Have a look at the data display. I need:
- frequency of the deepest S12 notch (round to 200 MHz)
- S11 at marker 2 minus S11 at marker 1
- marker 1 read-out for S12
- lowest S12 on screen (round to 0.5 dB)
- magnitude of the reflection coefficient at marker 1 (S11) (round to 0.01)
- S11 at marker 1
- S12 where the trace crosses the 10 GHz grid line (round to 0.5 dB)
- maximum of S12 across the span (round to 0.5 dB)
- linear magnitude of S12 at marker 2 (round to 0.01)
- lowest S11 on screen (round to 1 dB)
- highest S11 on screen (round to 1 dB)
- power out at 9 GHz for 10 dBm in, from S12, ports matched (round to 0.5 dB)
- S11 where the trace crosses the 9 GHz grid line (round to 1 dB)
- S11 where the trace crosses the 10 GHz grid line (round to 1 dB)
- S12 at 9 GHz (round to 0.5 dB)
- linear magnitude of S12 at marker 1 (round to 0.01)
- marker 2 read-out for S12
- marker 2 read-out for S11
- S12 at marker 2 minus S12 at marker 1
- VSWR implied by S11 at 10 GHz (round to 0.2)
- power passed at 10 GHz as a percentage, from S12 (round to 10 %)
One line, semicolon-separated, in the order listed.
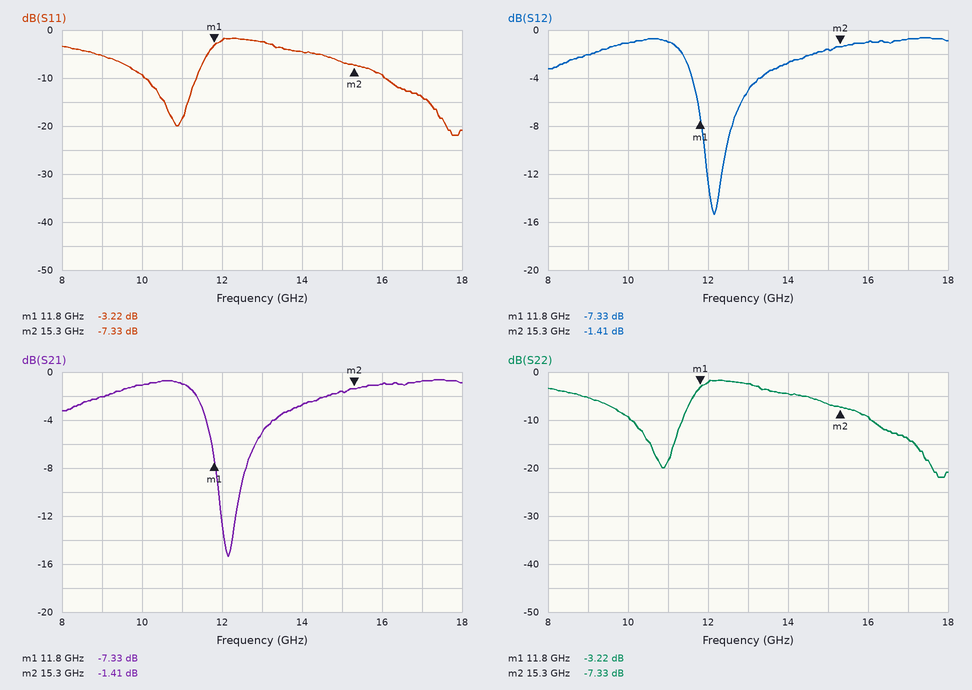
12.2 GHz; -4.11 dB; -7.33 dB; -15.5 dB; 0.69; -3.22 dB; -1.0 dB; -0.5 dB; 0.85; -22 dB; -2 dB; 8.0 dBm; -5 dB; -9 dB; -2.0 dB; 0.43; -1.41 dB; -7.33 dB; 5.92 dB; 2.0; 80 %
